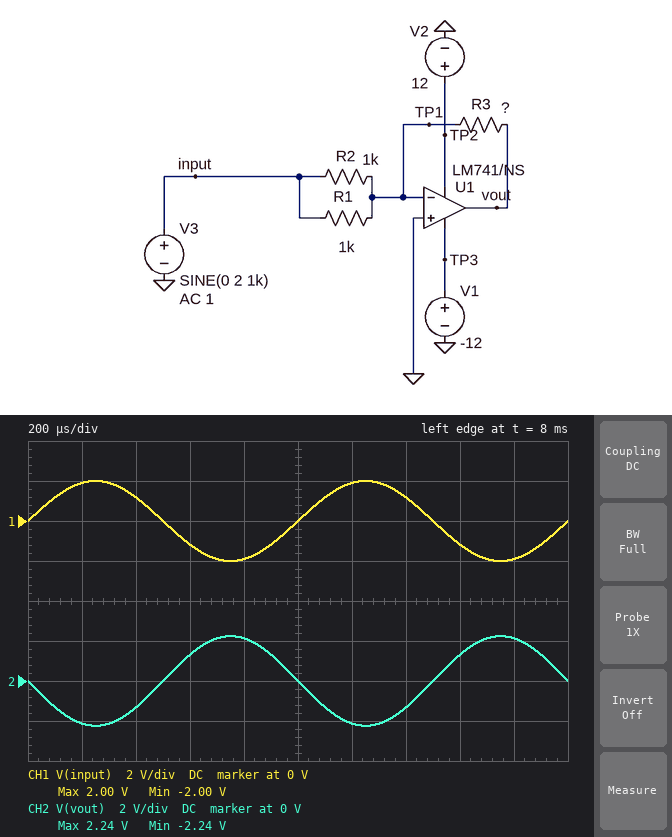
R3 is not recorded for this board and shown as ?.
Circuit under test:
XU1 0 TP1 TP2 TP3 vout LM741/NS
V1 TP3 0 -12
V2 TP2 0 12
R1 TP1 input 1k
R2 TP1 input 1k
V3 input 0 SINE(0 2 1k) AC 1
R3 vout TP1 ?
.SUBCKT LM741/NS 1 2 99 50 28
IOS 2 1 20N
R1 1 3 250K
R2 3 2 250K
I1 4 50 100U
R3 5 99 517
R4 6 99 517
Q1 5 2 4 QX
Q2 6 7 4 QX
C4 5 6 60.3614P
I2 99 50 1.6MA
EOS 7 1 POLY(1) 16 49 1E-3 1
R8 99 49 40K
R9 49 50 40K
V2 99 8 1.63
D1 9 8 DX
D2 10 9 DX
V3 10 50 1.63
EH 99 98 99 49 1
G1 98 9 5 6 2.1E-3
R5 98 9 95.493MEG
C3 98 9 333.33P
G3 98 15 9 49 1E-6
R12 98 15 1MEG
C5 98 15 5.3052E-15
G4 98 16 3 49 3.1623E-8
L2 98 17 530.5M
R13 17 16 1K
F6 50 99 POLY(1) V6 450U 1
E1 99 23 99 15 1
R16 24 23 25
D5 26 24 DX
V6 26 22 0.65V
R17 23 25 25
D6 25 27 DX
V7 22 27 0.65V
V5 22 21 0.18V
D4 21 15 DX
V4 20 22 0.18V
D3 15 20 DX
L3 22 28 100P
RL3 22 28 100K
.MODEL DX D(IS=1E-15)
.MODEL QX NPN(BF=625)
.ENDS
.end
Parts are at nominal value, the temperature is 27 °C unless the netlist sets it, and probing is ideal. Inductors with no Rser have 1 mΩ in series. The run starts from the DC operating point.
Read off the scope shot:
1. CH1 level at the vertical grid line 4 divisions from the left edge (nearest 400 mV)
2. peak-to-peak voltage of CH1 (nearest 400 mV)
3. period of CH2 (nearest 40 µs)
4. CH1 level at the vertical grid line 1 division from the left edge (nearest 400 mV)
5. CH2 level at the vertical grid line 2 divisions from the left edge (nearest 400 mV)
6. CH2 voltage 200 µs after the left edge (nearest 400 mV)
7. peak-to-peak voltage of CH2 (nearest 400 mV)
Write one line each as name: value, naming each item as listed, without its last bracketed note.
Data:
CH1 level at the vertical grid line 4 divisions from the left edge: -2.0 V
peak-to-peak voltage of CH1: 4.0 V
period of CH2: 1.00 ms
CH1 level at the vertical grid line 1 division from the left edge: 2.0 V
CH2 level at the vertical grid line 2 divisions from the left edge: -1.2 V
CH2 voltage 200 µs after the left edge: -2.0 V
peak-to-peak voltage of CH2: 4.4 V
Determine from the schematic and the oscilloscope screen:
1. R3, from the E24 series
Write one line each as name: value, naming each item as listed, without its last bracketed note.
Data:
R3, from the E24 series: 560 Ω
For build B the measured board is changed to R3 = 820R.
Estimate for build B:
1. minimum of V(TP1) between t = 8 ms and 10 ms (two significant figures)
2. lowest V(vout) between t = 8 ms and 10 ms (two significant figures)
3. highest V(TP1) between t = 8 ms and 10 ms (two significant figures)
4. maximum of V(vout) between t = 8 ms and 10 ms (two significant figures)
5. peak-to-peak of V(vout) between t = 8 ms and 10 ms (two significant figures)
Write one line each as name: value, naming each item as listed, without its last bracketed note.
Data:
minimum of V(TP1) between t = 8 ms and 10 ms: -3.0 mV
lowest V(vout) between t = 8 ms and 10 ms: -3.3 V
highest V(TP1) between t = 8 ms and 10 ms: 5.0 mV
maximum of V(vout) between t = 8 ms and 10 ms: 3.3 V
peak-to-peak of V(vout) between t = 8 ms and 10 ms: 6.6 V
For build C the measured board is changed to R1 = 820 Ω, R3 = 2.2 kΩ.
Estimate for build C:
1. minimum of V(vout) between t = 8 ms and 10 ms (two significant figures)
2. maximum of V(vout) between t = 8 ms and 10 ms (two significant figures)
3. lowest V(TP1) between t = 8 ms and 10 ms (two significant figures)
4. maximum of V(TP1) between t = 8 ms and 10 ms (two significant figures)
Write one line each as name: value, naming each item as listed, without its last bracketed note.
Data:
minimum of V(vout) between t = 8 ms and 10 ms: -9.8 V
maximum of V(vout) between t = 8 ms and 10 ms: 9.8 V
lowest V(TP1) between t = 8 ms and 10 ms: -9.7 mV
maximum of V(TP1) between t = 8 ms and 10 ms: 12 mV
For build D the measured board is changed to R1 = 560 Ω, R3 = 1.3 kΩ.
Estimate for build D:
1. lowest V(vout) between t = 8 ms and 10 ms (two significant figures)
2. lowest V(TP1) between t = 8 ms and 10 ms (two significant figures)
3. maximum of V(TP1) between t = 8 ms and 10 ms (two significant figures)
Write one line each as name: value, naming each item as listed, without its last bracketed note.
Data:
lowest V(vout) between t = 8 ms and 10 ms: -7.2 V
lowest V(TP1) between t = 8 ms and 10 ms: -7.3 mV
maximum of V(TP1) between t = 8 ms and 10 ms: 9.3 mV
